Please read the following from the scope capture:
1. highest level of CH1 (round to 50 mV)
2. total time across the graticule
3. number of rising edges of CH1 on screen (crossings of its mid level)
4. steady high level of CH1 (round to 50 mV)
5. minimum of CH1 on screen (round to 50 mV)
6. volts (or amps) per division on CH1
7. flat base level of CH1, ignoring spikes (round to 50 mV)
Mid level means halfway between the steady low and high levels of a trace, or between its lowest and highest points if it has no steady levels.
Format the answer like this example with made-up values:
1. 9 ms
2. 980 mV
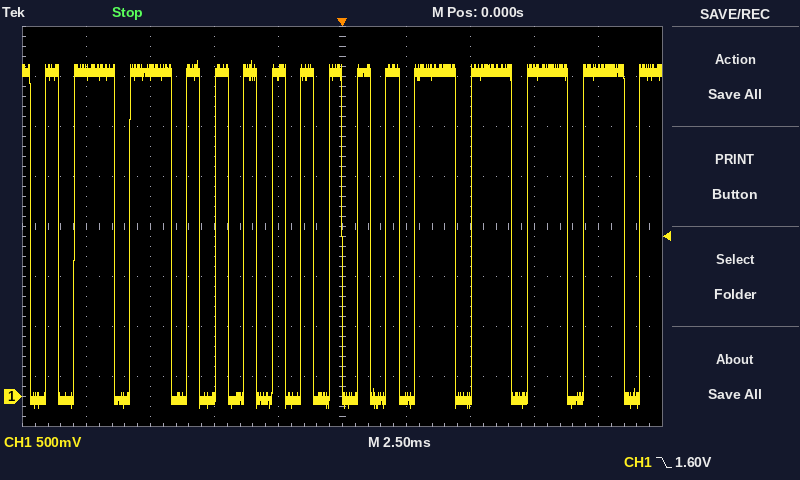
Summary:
1. 3.35 V
2. 25 ms
3. 16
4. 3.25 V
5. -100 mV
6. 500 mV
7. -50 mV
